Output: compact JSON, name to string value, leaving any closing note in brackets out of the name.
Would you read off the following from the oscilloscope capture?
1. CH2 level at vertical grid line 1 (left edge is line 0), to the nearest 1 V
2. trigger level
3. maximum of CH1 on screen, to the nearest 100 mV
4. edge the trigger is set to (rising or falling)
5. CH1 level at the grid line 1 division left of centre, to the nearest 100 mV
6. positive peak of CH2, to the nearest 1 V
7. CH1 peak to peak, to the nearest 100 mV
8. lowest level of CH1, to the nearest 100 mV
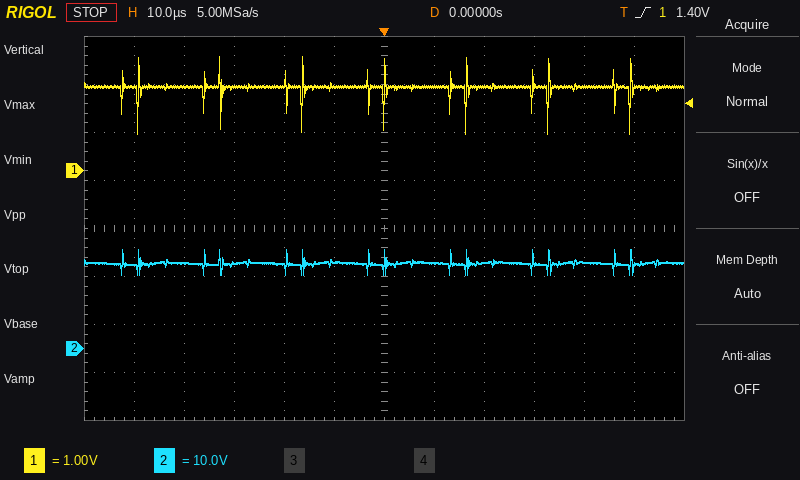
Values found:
{"CH2 level at vertical grid line 1 (left edge is line 0), to the nearest 1 V": "17 V", "trigger level": "1.40 V", "maximum of CH1 on screen, to the nearest 100 mV": "2.4 V", "edge the trigger is set to": "rising", "CH1 level at the grid line 1 division left of centre, to the nearest 100 mV": "1.8 V", "positive peak of CH2, to the nearest 1 V": "21 V", "CH1 peak to peak, to the nearest 100 mV": "1.6 V", "lowest level of CH1, to the nearest 100 mV": "800 mV"}
